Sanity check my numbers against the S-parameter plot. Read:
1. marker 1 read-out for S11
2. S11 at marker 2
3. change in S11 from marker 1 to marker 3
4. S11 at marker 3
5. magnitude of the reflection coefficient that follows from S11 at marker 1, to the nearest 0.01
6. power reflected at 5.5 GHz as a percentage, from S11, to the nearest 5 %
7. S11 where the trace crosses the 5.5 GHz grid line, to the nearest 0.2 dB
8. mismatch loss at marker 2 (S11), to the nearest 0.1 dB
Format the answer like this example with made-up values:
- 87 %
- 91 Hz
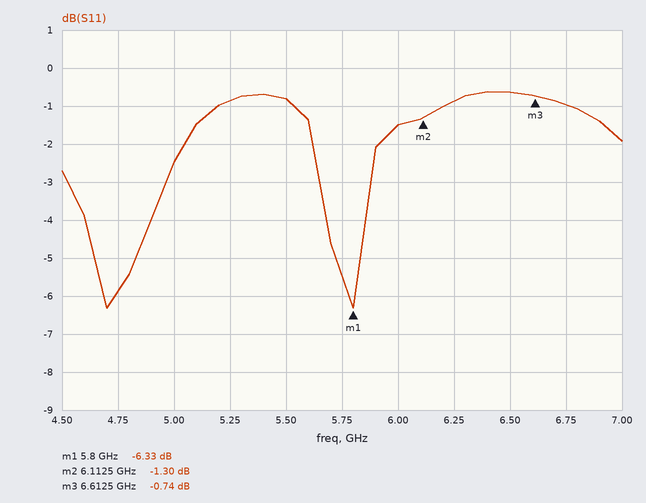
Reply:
- -6.33 dB
- -1.30 dB
- 5.59 dB
- -0.74 dB
- 0.48
- 85 %
- -0.8 dB
- 5.9 dB
